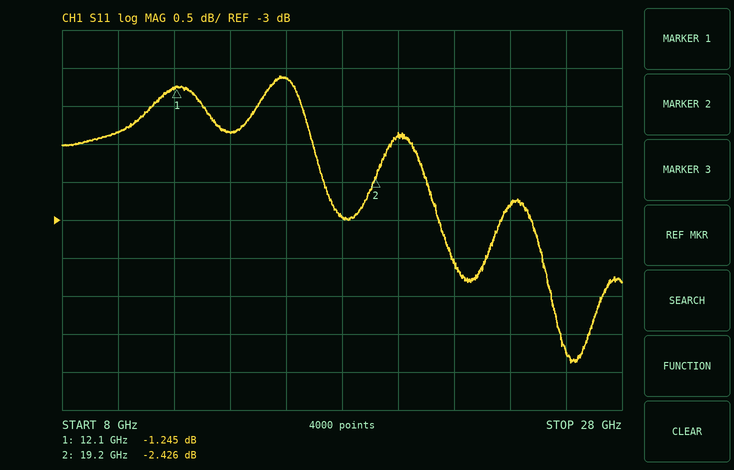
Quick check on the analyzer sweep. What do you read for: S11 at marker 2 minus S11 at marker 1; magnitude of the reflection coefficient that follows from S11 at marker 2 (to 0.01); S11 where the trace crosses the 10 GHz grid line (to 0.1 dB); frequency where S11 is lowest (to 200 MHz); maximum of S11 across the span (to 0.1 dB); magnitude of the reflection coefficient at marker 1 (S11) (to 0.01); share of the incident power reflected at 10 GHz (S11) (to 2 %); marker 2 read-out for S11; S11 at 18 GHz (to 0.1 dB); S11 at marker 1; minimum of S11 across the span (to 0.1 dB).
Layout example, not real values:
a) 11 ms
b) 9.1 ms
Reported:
a) -1.181 dB
b) 0.76
c) -1.8 dB
d) 26.2 GHz
e) -1.1 dB
f) 0.87
g) 66 %
h) -2.426 dB
i) -3.0 dB
j) -1.245 dB
k) -4.9 dB
